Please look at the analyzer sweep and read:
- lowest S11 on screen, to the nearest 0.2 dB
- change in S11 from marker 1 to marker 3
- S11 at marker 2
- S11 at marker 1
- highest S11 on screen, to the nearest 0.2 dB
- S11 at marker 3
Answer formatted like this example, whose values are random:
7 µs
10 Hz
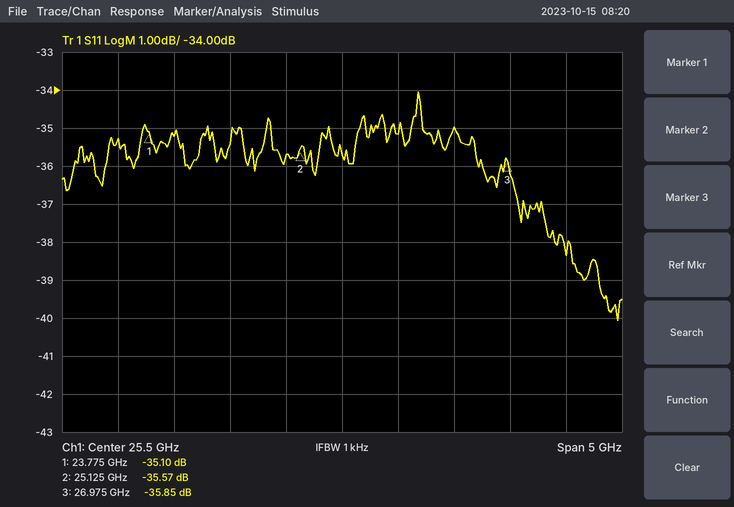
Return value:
-40.0 dB
-0.75 dB
-35.57 dB
-35.10 dB
-34.0 dB
-35.85 dB
